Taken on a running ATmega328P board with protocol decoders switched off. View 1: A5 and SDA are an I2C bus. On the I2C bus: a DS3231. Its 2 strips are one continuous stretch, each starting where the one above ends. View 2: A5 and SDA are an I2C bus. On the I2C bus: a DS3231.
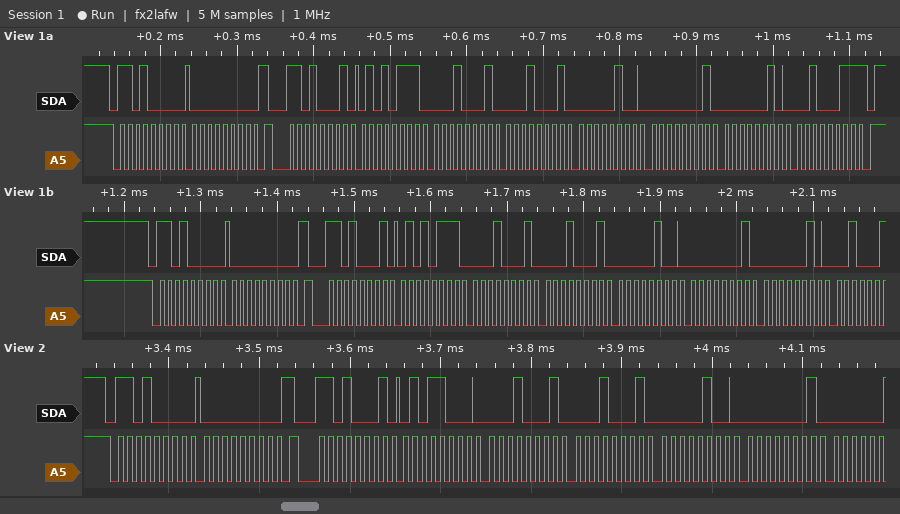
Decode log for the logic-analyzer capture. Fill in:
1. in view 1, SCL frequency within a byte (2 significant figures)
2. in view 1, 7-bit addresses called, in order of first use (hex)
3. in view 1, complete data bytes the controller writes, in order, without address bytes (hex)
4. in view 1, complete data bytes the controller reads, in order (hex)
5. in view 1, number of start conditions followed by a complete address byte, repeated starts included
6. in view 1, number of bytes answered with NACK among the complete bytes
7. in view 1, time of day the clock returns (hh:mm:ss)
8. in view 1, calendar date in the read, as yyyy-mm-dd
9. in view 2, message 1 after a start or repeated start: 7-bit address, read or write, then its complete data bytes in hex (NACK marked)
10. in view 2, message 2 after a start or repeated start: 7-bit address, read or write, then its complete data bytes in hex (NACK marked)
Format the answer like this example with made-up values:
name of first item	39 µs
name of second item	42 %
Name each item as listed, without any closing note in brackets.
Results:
in view 1, SCL frequency within a byte	100 kHz
in view 1, 7-bit addresses called, in order of first use	0x68
in view 1, complete data bytes the controller writes, in order, without address bytes	00 00
in view 1, complete data bytes the controller reads, in order	57 11 11 04 01 02 23 57 11 11 04 01 02
in view 1, number of start conditions followed by a complete address byte, repeated starts included	4
in view 1, number of bytes answered with NACK among the complete bytes	1
in view 1, time of day the clock returns	11:11:57
in view 1, calendar date in the read, as yyyy-mm-dd	2023-02-01
in view 2, message 1 after a start or repeated start: 7-bit address, read or write, then its complete data bytes in hex	0x68 write: 00
in view 2, message 2 after a start or repeated start: 7-bit address, read or write, then its complete data bytes in hex	0x68 read: 58 11 11 04 01
